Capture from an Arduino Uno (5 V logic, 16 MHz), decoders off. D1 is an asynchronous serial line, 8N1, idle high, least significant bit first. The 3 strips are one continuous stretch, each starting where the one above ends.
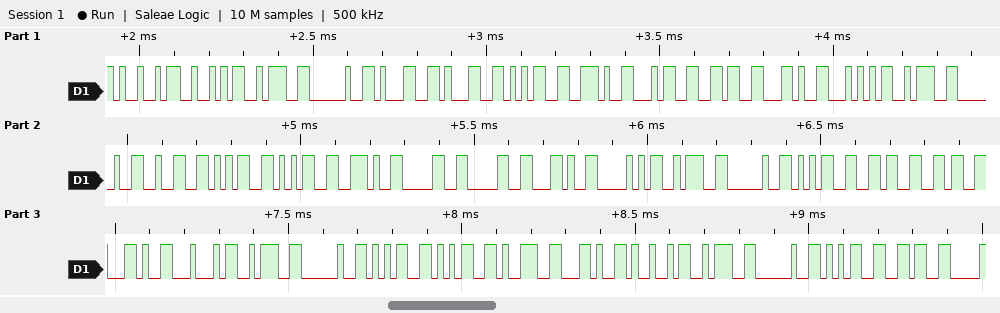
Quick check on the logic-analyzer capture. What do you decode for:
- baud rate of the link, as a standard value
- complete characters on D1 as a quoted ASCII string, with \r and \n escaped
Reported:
57600 baud
"IR: 115.46,T: 255.00,P: 566,D: 559,I: 56"
